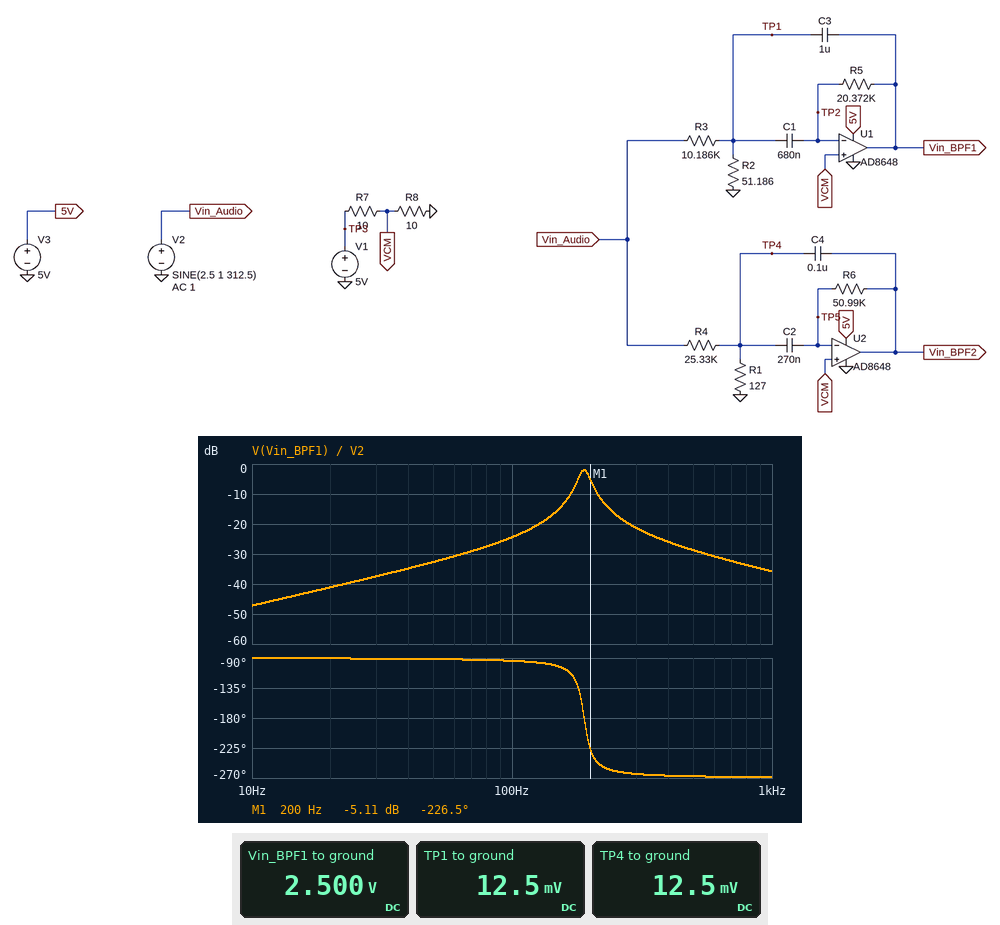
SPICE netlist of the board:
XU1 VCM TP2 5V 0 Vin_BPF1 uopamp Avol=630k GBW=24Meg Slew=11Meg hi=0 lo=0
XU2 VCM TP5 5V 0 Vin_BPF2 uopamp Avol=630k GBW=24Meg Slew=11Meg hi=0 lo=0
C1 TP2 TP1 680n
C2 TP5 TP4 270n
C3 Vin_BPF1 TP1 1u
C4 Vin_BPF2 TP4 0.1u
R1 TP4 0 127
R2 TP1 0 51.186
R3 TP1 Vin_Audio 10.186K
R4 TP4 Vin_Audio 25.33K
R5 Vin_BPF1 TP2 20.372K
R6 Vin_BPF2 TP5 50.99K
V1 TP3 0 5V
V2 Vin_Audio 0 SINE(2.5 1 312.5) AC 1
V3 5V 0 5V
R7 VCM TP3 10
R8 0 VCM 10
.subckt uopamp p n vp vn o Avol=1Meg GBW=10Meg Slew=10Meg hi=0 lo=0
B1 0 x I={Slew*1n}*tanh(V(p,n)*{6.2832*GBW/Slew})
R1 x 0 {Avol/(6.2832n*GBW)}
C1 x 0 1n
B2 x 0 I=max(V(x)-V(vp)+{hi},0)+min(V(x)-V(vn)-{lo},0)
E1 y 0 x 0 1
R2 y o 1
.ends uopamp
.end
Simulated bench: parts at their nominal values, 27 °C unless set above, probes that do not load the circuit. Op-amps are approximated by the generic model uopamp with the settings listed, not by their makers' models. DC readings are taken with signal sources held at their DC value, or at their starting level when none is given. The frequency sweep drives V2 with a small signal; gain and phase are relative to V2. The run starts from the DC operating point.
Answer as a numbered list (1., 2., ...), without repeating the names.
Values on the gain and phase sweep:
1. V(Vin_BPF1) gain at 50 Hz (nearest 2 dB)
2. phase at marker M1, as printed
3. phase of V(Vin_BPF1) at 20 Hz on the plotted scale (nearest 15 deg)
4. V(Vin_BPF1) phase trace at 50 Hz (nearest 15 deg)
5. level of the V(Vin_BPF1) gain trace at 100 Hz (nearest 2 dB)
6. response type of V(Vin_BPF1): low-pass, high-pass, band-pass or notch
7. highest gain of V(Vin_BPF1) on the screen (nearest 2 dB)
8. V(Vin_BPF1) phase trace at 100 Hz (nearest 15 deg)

1. -32 dB
2. -226.5 deg
3. -90 deg
4. -90 deg
5. -24 dB
6. band-pass
7. -2 dB
8. -90 deg
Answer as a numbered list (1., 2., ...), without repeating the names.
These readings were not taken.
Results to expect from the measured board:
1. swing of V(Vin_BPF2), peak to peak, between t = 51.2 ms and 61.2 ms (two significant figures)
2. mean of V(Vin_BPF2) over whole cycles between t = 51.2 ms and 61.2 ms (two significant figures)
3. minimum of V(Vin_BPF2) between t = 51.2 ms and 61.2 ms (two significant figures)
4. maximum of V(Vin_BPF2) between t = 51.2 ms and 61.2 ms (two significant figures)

1. 790 mV
2. 2.5 V
3. 2.1 V
4. 2.9 V
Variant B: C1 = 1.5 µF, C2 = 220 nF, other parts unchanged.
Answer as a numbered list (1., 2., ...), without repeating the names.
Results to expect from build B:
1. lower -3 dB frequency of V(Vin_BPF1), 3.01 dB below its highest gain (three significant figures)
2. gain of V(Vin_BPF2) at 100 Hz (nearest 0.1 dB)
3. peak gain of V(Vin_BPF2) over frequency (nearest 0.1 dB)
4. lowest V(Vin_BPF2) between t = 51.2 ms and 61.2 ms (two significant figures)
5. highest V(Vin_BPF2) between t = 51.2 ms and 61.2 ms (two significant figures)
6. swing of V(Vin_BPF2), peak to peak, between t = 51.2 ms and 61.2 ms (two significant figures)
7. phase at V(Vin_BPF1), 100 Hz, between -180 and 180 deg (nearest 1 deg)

1. 121 Hz
2. -28.6 dB
3. 2.8 dB
4. 2.3 V
5. 2.7 V
6. 480 mV
7. -102 deg
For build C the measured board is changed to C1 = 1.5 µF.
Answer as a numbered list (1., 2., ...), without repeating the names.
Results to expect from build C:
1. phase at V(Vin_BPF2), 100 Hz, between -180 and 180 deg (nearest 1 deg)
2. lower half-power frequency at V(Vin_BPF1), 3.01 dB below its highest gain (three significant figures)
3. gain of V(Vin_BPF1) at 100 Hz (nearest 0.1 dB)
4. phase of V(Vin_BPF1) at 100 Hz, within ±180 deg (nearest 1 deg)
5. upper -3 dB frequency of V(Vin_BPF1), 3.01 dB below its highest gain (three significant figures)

1. -92 deg
2. 121 Hz
3. -12.3 dB
4. -102 deg
5. 134 Hz
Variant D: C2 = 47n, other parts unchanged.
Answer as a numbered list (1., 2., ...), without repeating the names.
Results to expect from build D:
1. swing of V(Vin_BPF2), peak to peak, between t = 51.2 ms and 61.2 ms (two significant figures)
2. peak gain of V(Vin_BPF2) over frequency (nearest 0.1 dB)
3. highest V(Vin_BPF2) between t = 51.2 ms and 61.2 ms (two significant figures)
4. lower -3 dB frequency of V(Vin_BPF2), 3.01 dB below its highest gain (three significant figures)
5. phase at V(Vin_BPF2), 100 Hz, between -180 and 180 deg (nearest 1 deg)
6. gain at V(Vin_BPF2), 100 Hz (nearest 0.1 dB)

1. 53 mV
2. -3.8 dB
3. 2.5 V
4. 867 Hz
5. -91 deg
6. -42.4 dB
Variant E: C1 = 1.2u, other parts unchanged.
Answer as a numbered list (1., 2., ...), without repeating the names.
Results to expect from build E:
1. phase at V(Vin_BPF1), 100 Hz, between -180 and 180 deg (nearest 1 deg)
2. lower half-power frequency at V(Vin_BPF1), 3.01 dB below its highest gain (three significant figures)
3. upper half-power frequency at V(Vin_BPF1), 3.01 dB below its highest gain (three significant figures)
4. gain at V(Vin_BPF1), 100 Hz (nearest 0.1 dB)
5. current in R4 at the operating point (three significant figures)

1. -98 deg
2. 136 Hz
3. 150 Hz
4. -16.5 dB
5. 98.2 µA
